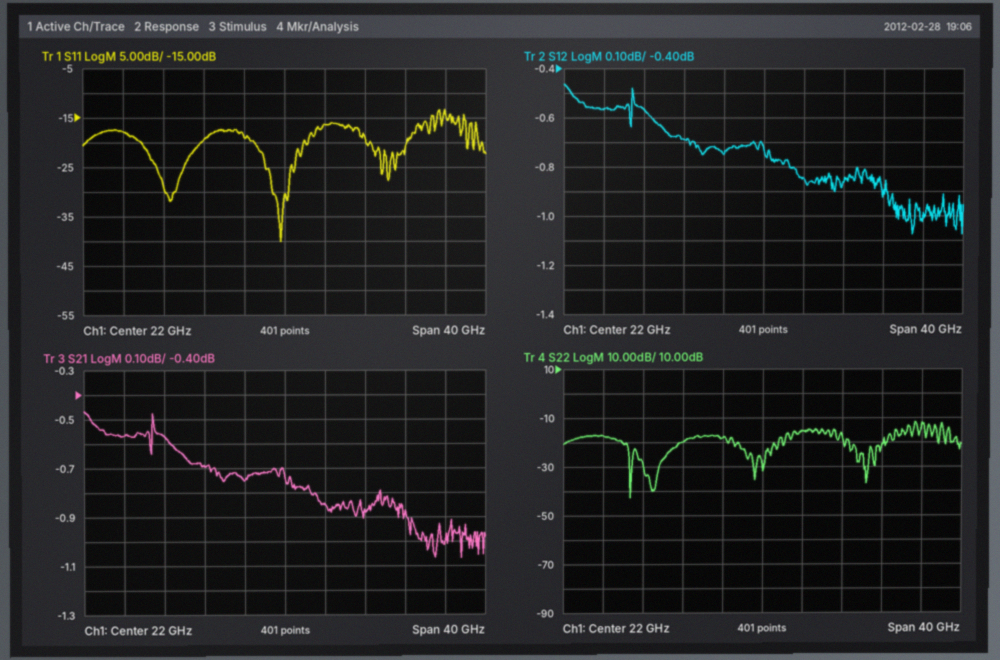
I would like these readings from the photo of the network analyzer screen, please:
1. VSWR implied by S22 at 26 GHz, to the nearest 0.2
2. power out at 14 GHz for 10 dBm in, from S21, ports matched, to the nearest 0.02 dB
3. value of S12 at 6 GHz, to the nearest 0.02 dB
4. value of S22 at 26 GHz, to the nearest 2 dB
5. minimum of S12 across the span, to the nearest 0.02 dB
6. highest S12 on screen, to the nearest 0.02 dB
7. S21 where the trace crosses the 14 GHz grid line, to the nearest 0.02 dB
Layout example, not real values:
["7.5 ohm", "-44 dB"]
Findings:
["1.4", "9.30 dBm", "-0.56 dB", "-16 dB", "-1.08 dB", "-0.46 dB", "-0.70 dB"]
